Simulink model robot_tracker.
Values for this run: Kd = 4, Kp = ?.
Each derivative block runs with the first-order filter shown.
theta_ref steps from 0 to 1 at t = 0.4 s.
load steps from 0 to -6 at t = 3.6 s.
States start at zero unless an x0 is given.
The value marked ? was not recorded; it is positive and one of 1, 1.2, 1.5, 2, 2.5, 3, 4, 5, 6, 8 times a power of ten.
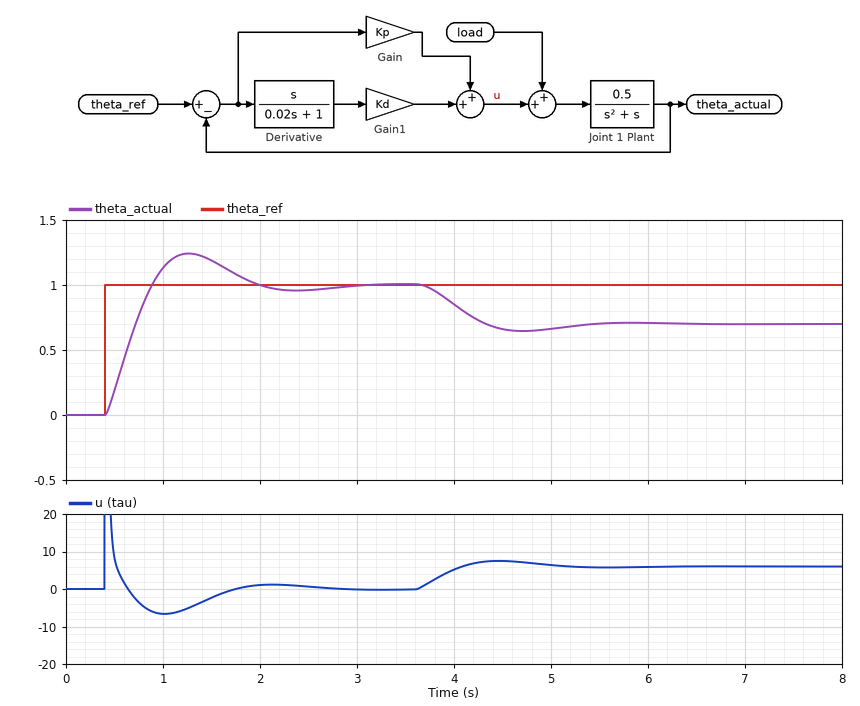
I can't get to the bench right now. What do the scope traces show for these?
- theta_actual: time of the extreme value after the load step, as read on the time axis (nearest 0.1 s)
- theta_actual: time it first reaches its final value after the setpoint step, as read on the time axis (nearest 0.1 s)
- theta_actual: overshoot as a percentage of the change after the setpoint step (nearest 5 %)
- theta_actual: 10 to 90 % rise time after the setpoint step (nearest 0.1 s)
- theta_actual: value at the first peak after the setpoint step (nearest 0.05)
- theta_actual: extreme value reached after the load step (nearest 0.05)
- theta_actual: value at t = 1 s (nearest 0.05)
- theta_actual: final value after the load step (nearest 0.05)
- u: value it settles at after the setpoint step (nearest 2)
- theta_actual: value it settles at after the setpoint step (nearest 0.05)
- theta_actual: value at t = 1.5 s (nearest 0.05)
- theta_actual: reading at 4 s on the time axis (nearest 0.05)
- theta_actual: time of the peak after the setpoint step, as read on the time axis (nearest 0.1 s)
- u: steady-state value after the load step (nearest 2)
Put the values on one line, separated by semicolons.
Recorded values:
4.7 s; 0.9 s; 25 %; 0.4 s; 1.25; 0.65; 1.15; 0.70; 0; 1.00; 1.20; 0.85; 1.3 s; 6
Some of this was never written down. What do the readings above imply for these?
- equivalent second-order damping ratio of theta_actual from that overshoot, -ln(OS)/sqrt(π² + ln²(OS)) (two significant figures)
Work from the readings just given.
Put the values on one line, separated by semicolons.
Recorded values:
0.40
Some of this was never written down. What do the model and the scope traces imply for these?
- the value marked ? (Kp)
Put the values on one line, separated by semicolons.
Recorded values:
20
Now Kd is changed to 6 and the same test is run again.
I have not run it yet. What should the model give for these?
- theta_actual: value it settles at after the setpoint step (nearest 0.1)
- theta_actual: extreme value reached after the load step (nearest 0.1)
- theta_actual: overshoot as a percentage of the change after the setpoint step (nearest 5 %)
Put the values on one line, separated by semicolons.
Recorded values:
1.0; 0.7; 15 %
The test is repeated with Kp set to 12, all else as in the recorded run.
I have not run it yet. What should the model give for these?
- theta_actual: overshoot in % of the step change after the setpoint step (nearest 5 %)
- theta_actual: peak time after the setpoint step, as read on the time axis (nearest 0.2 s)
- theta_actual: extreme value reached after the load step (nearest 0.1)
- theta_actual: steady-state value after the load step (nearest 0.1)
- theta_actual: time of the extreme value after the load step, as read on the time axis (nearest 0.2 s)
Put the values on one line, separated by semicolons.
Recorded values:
15 %; 1.6 s; 0.5; 0.5; 5.2 s
